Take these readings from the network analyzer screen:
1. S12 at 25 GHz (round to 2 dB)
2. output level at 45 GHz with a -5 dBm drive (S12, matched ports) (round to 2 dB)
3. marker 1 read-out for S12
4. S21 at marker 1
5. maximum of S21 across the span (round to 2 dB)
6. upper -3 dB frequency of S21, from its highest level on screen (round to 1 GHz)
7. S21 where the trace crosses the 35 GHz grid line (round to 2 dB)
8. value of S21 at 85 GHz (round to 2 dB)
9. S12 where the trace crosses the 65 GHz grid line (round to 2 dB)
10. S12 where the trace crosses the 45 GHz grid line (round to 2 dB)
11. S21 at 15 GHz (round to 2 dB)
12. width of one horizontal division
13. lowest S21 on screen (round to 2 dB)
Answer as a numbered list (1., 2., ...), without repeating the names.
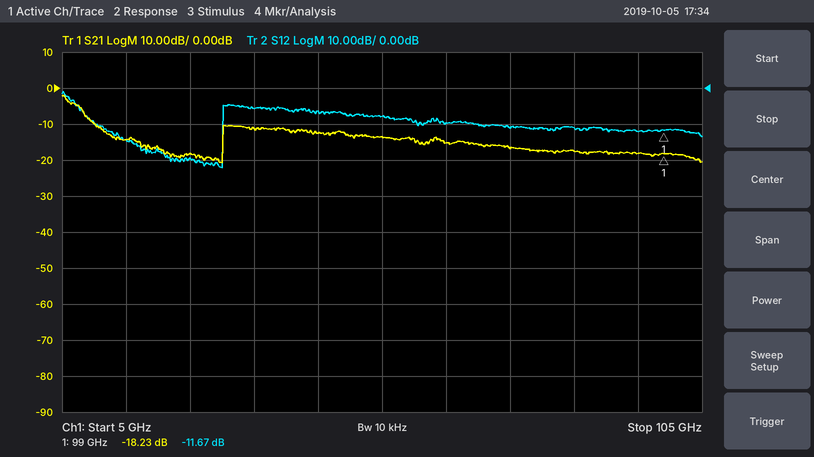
1. -20 dB
2. -12 dBm
3. -11.67 dB
4. -18.23 dB
5. -2 dB
6. 8 GHz
7. -12 dB
8. -18 dB
9. -10 dB
10. -6 dB
11. -14 dB
12. 10 GHz
13. -20 dB
